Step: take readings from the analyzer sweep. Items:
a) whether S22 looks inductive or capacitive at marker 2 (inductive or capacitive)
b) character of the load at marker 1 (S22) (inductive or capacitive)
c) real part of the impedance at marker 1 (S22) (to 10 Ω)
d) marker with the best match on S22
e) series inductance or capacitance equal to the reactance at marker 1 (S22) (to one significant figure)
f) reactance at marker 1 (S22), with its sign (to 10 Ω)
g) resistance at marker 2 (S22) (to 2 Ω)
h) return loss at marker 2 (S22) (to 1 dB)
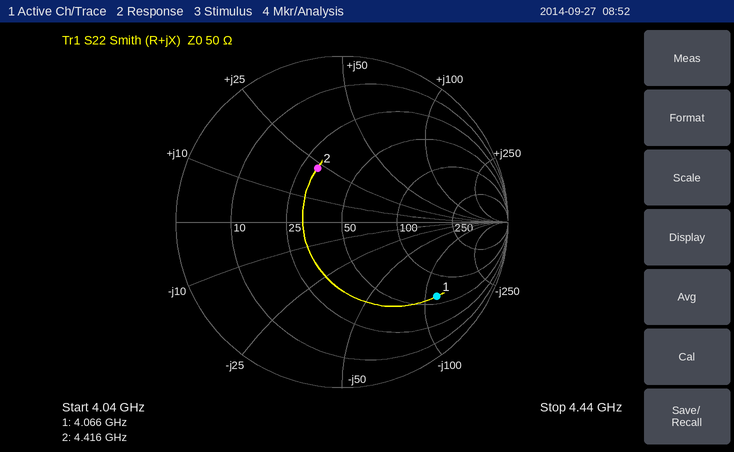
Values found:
inductive
capacitive
60 Ω
marker 2
300 fF
-120 Ω
30 Ω
9 dB
